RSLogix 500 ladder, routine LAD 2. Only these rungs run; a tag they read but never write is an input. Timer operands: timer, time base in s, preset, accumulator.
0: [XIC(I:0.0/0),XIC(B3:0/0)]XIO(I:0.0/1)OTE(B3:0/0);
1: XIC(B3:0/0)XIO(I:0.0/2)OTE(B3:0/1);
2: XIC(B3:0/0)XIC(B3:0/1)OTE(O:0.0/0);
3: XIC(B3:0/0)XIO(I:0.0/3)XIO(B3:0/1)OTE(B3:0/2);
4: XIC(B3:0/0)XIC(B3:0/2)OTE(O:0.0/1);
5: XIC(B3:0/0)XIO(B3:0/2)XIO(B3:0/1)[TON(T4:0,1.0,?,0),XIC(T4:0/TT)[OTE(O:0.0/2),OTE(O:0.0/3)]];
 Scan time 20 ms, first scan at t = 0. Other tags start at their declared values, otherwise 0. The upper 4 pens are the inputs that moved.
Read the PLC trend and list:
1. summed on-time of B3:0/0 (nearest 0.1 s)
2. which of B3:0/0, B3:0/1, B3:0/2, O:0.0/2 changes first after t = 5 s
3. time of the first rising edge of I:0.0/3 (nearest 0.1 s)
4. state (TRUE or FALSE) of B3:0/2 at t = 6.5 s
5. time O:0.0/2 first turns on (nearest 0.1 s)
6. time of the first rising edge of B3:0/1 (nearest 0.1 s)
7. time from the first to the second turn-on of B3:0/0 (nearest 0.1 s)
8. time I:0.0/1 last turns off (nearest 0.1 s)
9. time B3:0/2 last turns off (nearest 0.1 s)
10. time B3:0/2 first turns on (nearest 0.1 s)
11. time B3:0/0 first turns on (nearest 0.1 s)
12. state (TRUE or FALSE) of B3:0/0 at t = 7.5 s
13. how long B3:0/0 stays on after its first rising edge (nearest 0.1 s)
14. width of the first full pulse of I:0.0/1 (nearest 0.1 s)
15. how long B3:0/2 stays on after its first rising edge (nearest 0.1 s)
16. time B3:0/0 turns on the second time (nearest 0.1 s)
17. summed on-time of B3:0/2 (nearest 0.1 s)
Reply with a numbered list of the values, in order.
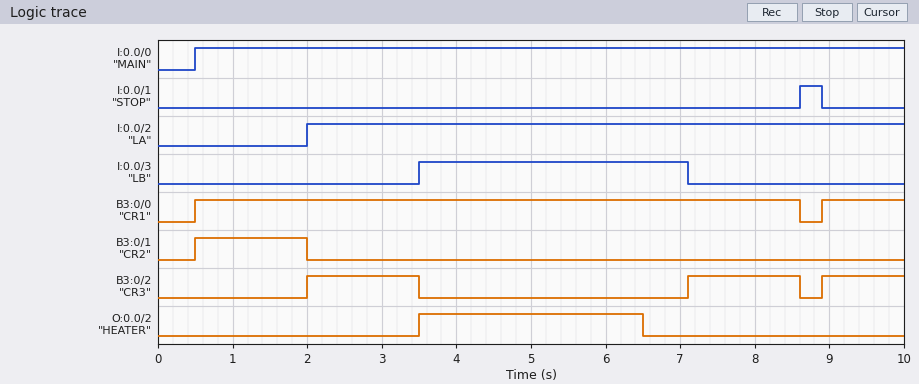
1. 9.2 s
2. O:0.0/2
3. 3.5 s
4. FALSE
5. 3.5 s
6. 0.5 s
7. 8.4 s
8. 8.9 s
9. 8.6 s
10. 2.0 s
11. 0.5 s
12. TRUE
13. 8.1 s
14. 0.3 s
15. 1.5 s
16. 8.9 s
17. 4.1 s
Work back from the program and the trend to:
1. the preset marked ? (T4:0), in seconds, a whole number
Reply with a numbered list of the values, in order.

1. 3 s
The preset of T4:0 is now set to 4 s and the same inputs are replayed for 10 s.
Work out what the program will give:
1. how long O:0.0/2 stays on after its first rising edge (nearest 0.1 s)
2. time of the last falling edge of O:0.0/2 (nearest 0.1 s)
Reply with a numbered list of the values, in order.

1. 3.6 s
2. 7.1 s
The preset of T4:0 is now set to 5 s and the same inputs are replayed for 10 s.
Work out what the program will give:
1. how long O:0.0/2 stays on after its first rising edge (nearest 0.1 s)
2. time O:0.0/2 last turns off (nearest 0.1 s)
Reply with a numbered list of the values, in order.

1. 3.6 s
2. 7.1 s
